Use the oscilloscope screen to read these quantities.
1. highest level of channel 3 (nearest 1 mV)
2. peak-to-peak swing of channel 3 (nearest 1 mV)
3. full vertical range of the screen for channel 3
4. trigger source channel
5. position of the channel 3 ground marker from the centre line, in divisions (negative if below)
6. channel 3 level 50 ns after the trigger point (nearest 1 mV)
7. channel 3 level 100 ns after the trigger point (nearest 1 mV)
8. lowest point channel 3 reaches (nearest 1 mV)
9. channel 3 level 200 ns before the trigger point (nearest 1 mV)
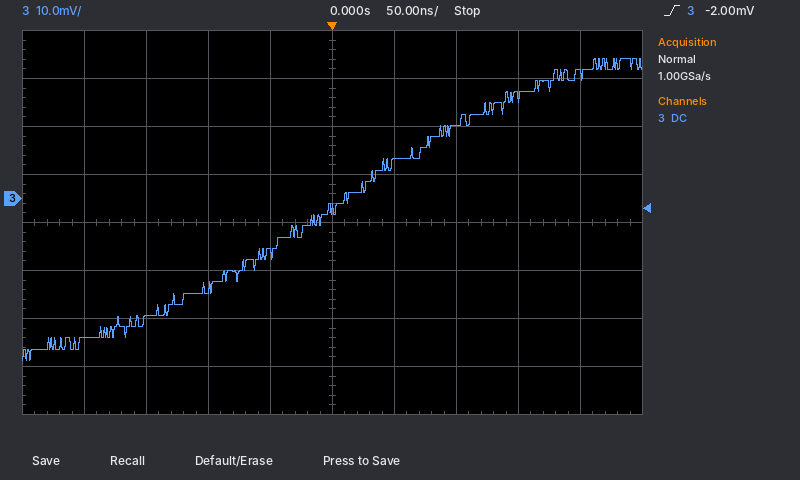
29 mV
63 mV
80 mV
channel 3
+0.5 div
7 mV
15 mV
-34 mV
-29 mV
